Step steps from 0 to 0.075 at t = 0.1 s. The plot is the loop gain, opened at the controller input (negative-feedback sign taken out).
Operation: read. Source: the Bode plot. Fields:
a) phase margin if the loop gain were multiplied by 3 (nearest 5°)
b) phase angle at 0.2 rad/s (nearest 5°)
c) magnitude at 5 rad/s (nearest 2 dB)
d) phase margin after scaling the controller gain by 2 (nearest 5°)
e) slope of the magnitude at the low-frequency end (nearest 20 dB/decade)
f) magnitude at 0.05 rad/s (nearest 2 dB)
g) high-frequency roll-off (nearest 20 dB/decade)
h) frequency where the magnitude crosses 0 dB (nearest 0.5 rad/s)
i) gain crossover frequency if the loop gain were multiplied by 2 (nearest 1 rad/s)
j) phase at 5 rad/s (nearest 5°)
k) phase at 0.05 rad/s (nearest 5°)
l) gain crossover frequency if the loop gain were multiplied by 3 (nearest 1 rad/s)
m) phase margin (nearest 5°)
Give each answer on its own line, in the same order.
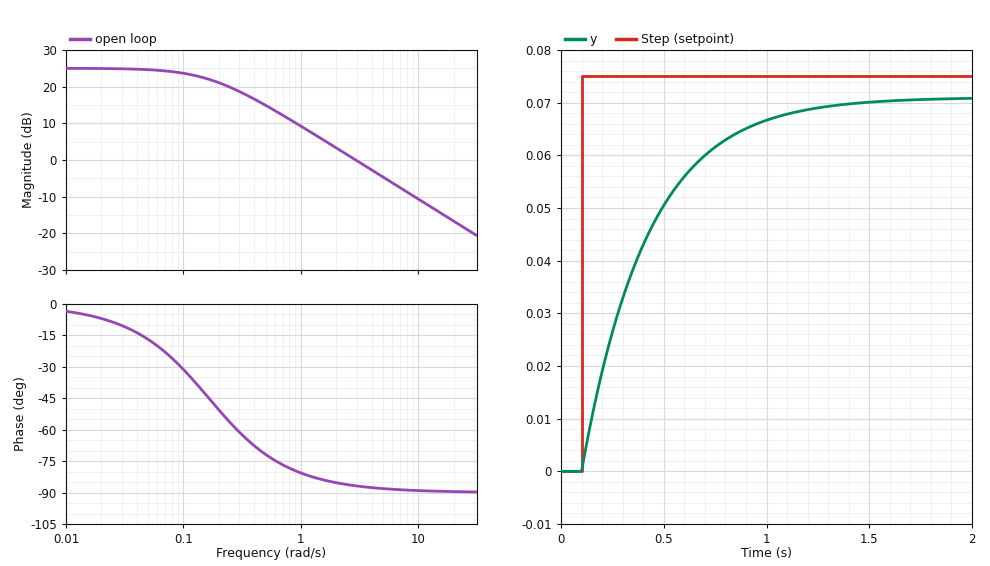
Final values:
90°
-50°
-4 dB
90°
0 dB/decade
24 dB
-20 dB/decade
3.0 rad/s
6 rad/s
-90°
-15°
9 rad/s
95°
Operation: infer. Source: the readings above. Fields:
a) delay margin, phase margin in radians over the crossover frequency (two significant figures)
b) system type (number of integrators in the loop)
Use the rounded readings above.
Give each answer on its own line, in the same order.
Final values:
0.55 s
0
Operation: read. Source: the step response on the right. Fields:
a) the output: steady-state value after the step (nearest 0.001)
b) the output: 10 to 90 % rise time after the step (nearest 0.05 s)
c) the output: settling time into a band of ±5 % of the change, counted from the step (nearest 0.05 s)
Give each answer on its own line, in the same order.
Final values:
0.071
0.70 s
0.95 s
